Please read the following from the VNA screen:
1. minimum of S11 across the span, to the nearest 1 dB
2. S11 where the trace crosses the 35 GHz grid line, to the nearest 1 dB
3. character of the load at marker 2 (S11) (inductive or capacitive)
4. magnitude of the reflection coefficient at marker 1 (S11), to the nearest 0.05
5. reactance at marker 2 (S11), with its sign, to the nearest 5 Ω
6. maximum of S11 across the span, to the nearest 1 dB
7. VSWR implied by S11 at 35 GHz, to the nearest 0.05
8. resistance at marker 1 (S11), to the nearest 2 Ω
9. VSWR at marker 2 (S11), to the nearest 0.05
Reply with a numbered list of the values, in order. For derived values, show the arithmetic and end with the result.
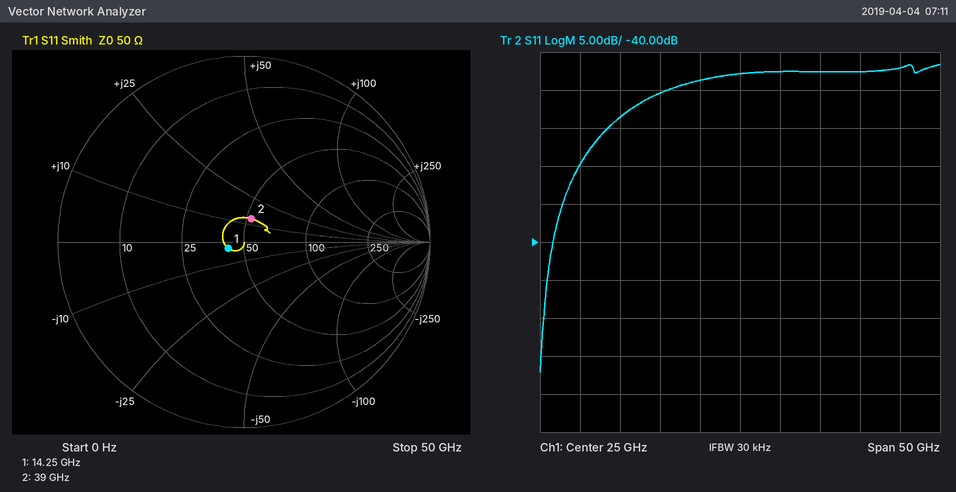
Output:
1. -57 dB
2. -18 dB
3. inductive
4. 0.10
5. +15 Ω
6. -17 dB
7. |Γ| = 10^(-18/20) = 0.1259; VSWR = (1 + 0.1259)/(1 − 0.1259) ≈ 1.29, so 1.30 to the nearest 0.05
8. 42 Ω
9. 1.30
